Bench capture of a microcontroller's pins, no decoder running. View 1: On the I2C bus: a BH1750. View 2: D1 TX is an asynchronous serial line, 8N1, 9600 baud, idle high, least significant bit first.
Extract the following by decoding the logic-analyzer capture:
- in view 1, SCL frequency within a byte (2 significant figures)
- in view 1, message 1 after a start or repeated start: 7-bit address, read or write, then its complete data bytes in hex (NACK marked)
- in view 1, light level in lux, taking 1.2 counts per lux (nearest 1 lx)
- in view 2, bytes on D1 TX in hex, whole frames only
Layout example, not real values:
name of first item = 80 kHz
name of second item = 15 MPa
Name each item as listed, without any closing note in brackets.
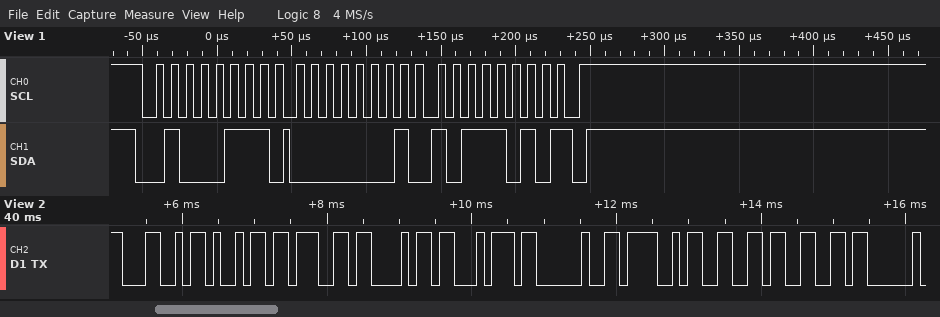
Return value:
in view 1, SCL frequency within a byte = 100 kHz
in view 1, message 1 after a start or repeated start: 7-bit address, read or write, then its complete data bytes in hex = 0x23 read: 01 BA NACK
in view 1, light level in lux, taking 1.2 counts per lux = 368 lx
in view 2, bytes on D1 TX in hex, whole frames only = 0x4C 0x69 0x67 0x68 0x74 0x20 0x4F 0x66 0x66
